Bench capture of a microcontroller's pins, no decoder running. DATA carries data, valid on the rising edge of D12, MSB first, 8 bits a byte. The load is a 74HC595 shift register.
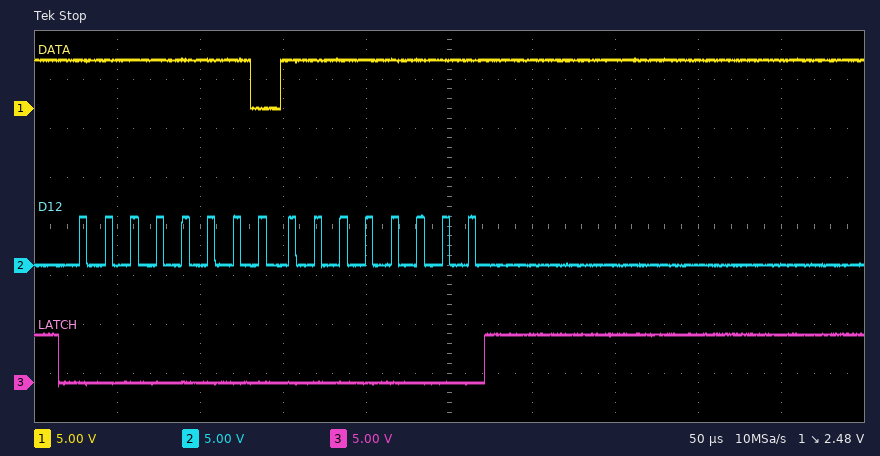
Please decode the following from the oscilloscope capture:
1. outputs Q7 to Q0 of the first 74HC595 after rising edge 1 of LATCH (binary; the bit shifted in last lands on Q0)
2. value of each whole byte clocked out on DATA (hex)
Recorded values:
11111111
FE FF
